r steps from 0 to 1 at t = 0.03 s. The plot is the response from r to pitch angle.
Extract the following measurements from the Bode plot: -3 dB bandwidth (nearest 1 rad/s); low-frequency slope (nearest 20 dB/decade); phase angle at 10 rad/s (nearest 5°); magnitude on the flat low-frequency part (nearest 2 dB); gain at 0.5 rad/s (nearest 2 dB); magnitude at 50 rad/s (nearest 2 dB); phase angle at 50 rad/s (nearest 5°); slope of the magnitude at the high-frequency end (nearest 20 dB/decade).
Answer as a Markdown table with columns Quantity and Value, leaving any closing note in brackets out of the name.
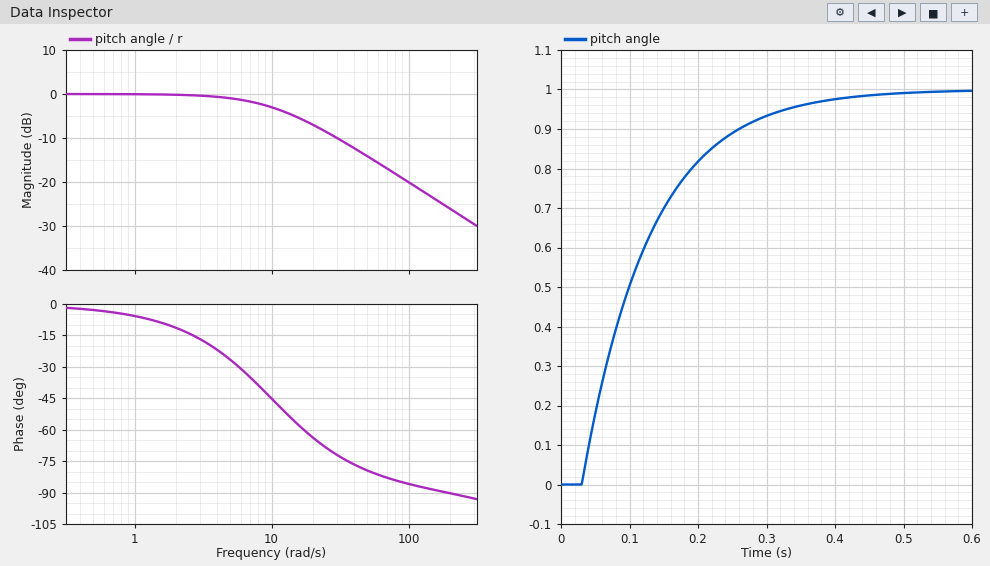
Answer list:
| Quantity | Value |
|---|---|
| -3 dB bandwidth | 10 rad/s |
| low-frequency slope | 0 dB/decade |
| phase angle at 10 rad/s | -45° |
| magnitude on the flat low-frequency part | 0 dB |
| gain at 0.5 rad/s | 0 dB |
| magnitude at 50 rad/s | -14 dB |
| phase angle at 50 rad/s | -80° |
| slope of the magnitude at the high-frequency end | -20 dB/decade |
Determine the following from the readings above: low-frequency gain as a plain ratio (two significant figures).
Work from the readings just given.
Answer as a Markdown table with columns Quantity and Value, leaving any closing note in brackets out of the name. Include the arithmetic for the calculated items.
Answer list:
| Quantity | Value |
|---|---|
| low-frequency gain as a plain ratio | 10^(0 / 20) = 1.0 |
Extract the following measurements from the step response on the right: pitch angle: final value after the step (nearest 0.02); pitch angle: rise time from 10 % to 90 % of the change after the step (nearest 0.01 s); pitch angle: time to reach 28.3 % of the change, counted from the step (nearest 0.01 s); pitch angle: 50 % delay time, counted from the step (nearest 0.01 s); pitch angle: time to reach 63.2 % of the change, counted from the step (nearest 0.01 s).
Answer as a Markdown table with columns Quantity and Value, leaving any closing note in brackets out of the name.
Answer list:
| Quantity | Value |
|---|---|
| pitch angle: final value after the step | 1.00 |
| pitch angle: rise time from 10 % to 90 % of the change after the step | 0.22 s |
| pitch angle: time to reach 28.3 % of the change, counted from the step | 0.03 s |
| pitch angle: 50 % delay time, counted from the step | 0.07 s |
| pitch angle: time to reach 63.2 % of the change, counted from the step | 0.10 s |
